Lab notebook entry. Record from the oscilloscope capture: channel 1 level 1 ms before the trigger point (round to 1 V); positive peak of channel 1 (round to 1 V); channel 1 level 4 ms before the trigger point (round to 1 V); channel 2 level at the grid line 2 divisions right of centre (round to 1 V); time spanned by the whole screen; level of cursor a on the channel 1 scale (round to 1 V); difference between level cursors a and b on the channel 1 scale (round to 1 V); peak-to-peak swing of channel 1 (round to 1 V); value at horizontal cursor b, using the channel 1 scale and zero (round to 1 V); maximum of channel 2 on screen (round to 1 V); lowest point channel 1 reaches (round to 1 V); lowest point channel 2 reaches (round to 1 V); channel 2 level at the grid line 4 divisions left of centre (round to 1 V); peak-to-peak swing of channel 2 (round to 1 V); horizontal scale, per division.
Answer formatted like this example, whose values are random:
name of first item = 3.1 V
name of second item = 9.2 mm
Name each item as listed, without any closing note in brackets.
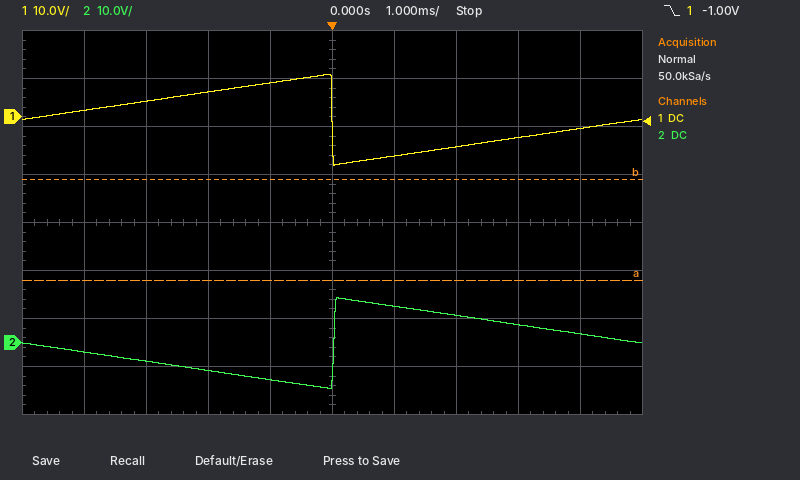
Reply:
channel 1 level 1 ms before the trigger point = 7 V
positive peak of channel 1 = 9 V
channel 1 level 4 ms before the trigger point = 1 V
channel 2 level at the grid line 2 divisions right of centre = 6 V
time spanned by the whole screen = 10 ms
level of cursor a on the channel 1 scale = -34 V
difference between level cursors a and b on the channel 1 scale = 21 V
peak-to-peak swing of channel 1 = 19 V
value at horizontal cursor b, using the channel 1 scale and zero = -13 V
maximum of channel 2 on screen = 9 V
lowest point channel 1 reaches = -10 V
lowest point channel 2 reaches = -10 V
channel 2 level at the grid line 4 divisions left of centre = -2 V
peak-to-peak swing of channel 2 = 19 V
horizontal scale, per division = 1 ms
